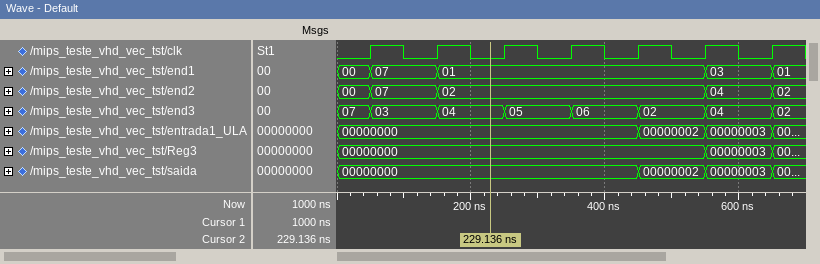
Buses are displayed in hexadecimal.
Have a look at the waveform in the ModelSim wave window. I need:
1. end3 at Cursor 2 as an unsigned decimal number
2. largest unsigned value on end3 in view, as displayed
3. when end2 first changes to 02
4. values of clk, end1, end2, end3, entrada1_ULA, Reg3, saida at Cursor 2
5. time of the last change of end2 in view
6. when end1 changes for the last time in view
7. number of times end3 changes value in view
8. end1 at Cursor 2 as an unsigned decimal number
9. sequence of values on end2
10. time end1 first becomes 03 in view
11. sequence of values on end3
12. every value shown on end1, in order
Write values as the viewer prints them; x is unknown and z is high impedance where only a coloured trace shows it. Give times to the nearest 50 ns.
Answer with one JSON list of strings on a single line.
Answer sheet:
["4", "07", "150 ns", "clk=0, end1=01, end2=02, end3=04, entrada1_ULA=00000000, Reg3=00000000, saida=00000000", "650 ns", "650 ns", "7", "1", "00, 07, 02, 04, 02", "550 ns", "07, 03, 04, 05, 06, 02, 04, 02", "00, 07, 01, 03, 01"]
